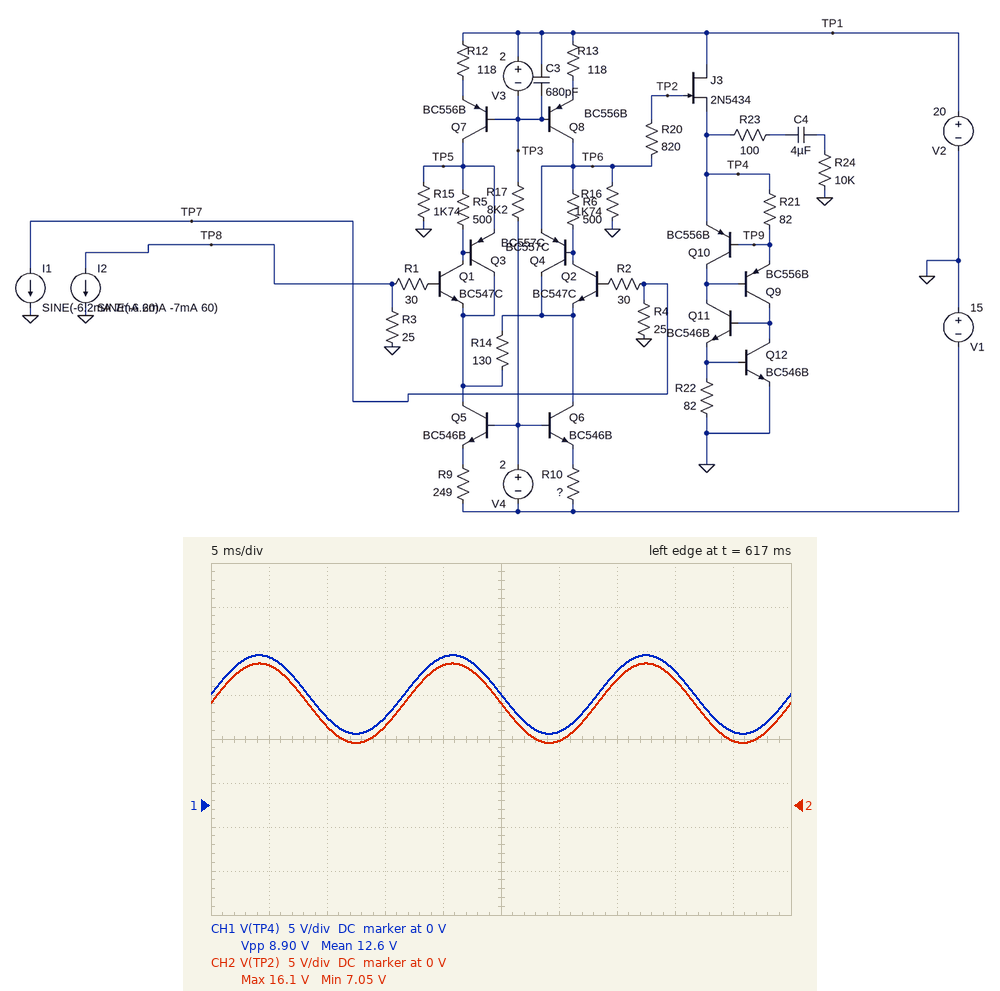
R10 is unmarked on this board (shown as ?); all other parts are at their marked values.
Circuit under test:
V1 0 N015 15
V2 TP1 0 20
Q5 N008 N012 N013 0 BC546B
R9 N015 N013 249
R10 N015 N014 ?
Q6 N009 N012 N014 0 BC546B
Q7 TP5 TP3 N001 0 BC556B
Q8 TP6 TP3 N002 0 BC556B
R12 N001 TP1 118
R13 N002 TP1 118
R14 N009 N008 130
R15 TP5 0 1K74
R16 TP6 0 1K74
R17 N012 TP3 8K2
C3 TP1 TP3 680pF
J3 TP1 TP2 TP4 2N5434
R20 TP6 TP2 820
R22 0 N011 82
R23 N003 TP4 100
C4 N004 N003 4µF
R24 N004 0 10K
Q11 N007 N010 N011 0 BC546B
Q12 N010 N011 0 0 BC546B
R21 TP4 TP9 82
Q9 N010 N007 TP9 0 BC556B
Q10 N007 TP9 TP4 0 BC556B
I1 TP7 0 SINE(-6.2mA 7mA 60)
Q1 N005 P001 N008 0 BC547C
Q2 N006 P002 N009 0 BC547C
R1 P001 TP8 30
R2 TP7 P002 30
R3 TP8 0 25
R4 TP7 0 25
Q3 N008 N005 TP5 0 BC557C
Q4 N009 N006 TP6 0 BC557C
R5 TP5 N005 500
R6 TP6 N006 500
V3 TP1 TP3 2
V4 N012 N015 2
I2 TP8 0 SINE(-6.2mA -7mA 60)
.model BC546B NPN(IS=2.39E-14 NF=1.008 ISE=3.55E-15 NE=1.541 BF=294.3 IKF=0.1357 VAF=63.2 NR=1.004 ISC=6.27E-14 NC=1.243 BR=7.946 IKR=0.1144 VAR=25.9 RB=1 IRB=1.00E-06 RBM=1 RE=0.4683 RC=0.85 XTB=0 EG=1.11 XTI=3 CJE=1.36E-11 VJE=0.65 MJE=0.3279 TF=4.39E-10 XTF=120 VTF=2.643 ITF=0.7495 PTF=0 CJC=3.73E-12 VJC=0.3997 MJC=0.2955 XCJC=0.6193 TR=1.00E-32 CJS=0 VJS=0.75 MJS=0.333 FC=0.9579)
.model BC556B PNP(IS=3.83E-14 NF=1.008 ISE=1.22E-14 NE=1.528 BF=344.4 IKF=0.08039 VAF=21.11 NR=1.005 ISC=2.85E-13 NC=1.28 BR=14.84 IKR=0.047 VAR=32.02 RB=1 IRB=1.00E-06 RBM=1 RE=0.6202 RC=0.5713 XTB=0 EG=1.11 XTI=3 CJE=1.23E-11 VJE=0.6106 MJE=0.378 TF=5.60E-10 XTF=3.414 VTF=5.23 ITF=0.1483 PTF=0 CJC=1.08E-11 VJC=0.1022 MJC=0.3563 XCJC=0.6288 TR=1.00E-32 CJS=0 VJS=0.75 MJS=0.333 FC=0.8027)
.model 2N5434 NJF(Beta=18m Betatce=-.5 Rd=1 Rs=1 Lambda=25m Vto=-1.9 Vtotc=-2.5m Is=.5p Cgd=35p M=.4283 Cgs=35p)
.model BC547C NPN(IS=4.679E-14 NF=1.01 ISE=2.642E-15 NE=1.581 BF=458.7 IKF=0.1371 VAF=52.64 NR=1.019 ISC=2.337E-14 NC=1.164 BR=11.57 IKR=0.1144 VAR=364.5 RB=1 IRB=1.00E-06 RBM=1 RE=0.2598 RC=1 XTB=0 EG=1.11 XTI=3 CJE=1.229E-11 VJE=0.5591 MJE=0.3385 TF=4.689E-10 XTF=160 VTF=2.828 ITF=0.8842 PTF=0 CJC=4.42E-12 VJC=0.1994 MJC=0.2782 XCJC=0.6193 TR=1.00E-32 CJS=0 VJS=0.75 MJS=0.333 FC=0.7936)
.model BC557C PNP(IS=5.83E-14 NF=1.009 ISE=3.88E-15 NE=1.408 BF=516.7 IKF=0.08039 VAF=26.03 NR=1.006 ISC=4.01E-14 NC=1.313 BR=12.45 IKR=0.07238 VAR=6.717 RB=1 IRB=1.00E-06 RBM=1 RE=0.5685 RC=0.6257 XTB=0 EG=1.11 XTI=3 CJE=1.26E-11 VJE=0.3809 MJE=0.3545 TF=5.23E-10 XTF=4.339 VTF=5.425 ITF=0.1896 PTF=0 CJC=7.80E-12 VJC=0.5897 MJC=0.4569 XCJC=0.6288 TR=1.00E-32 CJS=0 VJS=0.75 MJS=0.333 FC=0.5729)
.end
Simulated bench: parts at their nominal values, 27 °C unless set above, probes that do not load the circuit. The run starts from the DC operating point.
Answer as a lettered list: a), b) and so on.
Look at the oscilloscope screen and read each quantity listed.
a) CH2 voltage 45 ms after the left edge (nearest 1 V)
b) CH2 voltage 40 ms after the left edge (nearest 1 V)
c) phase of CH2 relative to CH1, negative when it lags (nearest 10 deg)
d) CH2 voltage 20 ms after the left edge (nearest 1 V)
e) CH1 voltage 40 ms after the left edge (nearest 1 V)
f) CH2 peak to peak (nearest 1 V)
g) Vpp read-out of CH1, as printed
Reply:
a) 7 V
b) 14 V
c) 0 deg
d) 16 V
e) 15 V
f) 9 V
g) 8.90 V
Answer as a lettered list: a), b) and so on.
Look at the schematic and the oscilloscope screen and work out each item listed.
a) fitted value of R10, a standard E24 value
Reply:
a) 300 Ω
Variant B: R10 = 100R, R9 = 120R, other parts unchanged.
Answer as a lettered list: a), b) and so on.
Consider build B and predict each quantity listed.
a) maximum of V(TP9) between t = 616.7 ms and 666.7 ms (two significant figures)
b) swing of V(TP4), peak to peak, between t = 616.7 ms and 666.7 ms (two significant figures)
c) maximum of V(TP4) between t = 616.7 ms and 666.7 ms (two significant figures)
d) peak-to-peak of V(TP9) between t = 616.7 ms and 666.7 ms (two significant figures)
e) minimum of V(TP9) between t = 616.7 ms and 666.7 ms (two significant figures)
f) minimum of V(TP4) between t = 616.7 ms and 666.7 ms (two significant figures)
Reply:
a) 1.2 V
b) 91 mV
c) 1.6 V
d) 47 mV
e) 1.1 V
f) 1.5 V
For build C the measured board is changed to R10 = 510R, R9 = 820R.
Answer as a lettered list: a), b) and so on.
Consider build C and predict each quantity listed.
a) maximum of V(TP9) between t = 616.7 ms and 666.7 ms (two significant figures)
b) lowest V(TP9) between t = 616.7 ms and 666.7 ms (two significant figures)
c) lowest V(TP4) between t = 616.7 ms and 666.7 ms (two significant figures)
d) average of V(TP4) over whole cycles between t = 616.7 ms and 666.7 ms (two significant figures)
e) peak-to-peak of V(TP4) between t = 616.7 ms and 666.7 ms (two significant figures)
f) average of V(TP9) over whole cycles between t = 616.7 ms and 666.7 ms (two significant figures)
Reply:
a) 19 V
b) 12 V
c) 13 V
d) 16 V
e) 6.5 V
f) 15 V
